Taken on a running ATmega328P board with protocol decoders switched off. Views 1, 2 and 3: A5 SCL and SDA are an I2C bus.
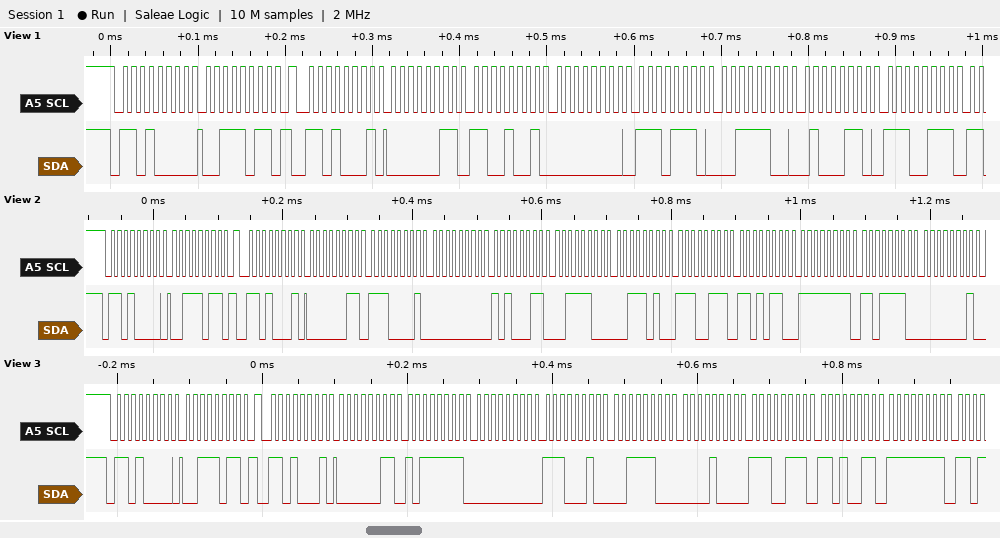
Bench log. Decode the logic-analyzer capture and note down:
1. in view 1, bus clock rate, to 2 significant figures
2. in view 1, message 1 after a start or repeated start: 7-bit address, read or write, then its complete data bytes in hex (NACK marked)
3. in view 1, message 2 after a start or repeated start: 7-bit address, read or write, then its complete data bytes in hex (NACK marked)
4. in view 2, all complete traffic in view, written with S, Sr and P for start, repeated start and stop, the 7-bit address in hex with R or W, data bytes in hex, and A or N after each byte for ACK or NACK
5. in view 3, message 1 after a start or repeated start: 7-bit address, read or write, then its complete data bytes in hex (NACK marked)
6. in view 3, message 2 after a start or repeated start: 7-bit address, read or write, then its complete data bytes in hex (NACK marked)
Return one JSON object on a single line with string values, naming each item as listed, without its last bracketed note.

{"in view 1, bus clock rate, to 2 significant figures": "100 kHz", "in view 1, message 1 after a start or repeated start: 7-bit address, read or write, then its complete data bytes in hex": "0x68 write: 3B", "in view 1, message 2 after a start or repeated start: 7-bit address, read or write, then its complete data bytes in hex": "0x68 read: 03 C9 00 EE 3C 46 E7", "in view 2, all complete traffic in view, written with S, Sr and P for start, repeated start and stop, the 7-bit address in hex with R or W, data bytes in hex, and A or N after each byte for ACK or NACK": "S 68W A 3B A Sr 68R A 03 A E1 A 00 A A3 A 3C A 3A A E7 A D6 A FF A DE A 01 A", "in view 3, message 1 after a start or repeated start: 7-bit address, read or write, then its complete data bytes in hex": "0x68 write: 3B", "in view 3, message 2 after a start or repeated start: 7-bit address, read or write, then its complete data bytes in hex": "0x68 read: 03 BF 00 E2 3C 08 E7 D3 FF"}
